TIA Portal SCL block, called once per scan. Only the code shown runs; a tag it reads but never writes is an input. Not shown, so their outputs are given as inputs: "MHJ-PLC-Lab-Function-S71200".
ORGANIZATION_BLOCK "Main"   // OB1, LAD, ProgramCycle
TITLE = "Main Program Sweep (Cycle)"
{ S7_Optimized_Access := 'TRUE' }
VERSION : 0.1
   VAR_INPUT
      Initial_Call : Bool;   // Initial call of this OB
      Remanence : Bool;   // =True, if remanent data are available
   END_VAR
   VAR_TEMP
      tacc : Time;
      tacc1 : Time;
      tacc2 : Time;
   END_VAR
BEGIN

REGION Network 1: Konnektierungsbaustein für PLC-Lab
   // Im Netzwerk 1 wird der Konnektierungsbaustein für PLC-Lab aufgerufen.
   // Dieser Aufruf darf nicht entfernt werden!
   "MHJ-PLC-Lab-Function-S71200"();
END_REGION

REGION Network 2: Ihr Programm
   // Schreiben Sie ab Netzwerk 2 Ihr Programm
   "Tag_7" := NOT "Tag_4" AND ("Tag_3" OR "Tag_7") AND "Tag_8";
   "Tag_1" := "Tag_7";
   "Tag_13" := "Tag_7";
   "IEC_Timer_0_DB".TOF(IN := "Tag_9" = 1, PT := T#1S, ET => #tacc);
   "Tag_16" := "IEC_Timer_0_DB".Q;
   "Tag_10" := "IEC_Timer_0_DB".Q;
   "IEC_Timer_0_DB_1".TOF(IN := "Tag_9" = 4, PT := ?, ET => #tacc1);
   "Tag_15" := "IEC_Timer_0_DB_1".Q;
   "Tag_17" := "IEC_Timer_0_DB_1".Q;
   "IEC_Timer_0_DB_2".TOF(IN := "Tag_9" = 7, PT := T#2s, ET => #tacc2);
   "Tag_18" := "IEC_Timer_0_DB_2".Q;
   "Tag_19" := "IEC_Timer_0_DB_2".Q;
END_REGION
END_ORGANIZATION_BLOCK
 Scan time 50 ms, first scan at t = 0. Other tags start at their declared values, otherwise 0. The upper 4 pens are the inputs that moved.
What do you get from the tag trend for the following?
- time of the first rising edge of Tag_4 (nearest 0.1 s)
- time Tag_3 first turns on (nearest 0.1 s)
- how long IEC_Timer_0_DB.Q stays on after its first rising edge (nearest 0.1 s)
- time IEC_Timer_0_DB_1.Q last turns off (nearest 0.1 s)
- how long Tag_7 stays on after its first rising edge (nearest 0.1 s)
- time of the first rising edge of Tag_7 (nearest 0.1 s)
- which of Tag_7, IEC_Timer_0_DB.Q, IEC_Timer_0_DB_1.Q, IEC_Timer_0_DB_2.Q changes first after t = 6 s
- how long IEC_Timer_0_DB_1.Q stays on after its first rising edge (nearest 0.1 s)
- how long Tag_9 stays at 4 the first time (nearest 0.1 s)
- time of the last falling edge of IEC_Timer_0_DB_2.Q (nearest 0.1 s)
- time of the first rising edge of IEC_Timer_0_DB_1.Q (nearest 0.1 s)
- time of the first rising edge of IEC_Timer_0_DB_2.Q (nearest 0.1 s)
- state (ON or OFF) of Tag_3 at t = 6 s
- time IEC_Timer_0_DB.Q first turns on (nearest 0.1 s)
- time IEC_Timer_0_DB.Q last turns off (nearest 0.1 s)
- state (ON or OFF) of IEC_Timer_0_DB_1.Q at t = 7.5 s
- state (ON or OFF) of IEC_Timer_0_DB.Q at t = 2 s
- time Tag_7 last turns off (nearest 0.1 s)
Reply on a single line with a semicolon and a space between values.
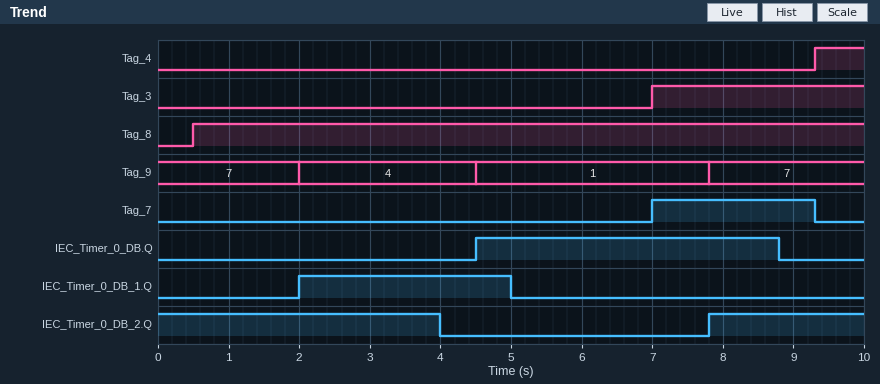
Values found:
9.3 s; 7.0 s; 4.3 s; 5.0 s; 2.3 s; 7.0 s; Tag_7; 3.0 s; 2.5 s; 4.0 s; 2.0 s; 7.8 s; OFF; 4.5 s; 8.8 s; OFF; OFF; 9.3 s
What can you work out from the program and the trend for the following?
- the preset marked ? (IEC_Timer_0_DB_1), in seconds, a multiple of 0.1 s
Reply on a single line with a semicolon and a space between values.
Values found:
0.5 s
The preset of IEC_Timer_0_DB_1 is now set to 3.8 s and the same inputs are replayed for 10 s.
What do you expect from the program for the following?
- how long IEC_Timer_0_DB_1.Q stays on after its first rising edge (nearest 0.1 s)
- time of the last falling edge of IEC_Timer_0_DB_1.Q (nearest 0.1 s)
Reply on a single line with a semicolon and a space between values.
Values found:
6.3 s; 8.3 s
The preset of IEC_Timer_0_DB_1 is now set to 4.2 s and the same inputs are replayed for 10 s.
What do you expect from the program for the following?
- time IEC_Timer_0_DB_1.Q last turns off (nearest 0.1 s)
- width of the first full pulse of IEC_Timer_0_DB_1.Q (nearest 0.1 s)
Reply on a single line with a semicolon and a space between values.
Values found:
8.7 s; 6.7 s
